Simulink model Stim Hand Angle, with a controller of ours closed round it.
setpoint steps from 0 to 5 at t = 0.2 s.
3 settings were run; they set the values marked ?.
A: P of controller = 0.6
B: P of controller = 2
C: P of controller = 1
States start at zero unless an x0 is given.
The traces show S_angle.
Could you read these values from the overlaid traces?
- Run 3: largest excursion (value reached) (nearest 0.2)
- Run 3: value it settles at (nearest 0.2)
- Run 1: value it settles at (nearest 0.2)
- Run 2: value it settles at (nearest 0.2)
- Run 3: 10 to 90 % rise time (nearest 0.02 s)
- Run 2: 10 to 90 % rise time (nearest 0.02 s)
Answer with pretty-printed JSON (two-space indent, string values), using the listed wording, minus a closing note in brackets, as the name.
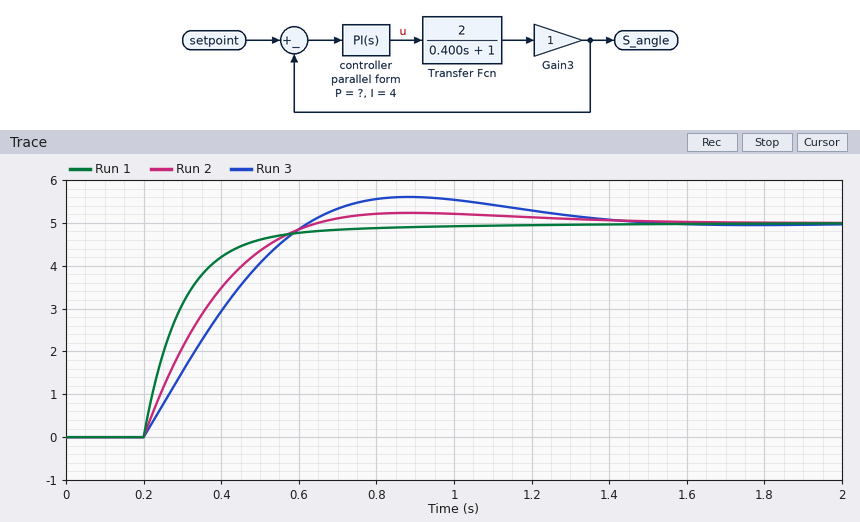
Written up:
{
  "Run 3: largest excursion (value reached)": "5.6",
  "Run 3: value it settles at": "5.0",
  "Run 1: value it settles at": "5.0",
  "Run 2: value it settles at": "5.0",
  "Run 3: 10 to 90 % rise time": "0.32 s",
  "Run 2: 10 to 90 % rise time": "0.30 s"
}
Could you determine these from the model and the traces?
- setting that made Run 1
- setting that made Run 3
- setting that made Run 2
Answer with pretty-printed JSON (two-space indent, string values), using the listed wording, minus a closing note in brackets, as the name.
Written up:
{
  "setting that made Run 1": "B",
  "setting that made Run 3": "A",
  "setting that made Run 2": "C"
}
